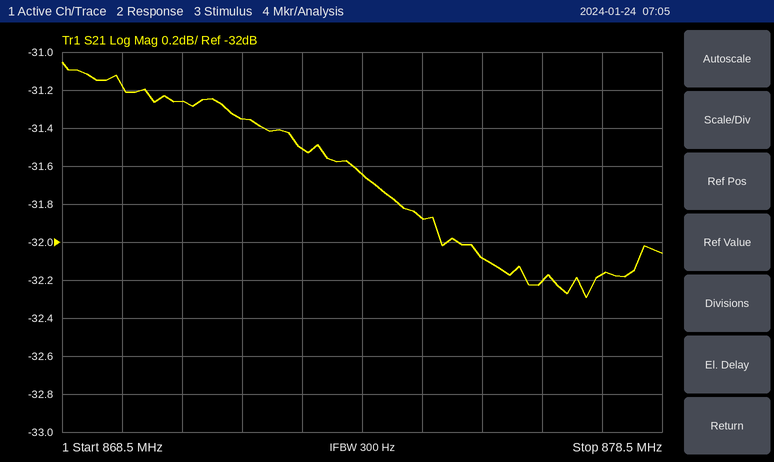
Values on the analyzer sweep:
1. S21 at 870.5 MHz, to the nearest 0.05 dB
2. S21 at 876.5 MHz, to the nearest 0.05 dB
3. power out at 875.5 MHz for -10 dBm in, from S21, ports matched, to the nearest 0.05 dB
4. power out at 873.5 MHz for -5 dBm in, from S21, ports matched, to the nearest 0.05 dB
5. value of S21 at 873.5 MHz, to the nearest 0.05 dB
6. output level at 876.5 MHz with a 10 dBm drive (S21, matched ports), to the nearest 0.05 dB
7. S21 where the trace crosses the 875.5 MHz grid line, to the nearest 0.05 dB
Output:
-31.25 dB
-32.20 dB
-42.10 dBm
-36.65 dBm
-31.65 dB
-22.20 dBm
-32.10 dB
